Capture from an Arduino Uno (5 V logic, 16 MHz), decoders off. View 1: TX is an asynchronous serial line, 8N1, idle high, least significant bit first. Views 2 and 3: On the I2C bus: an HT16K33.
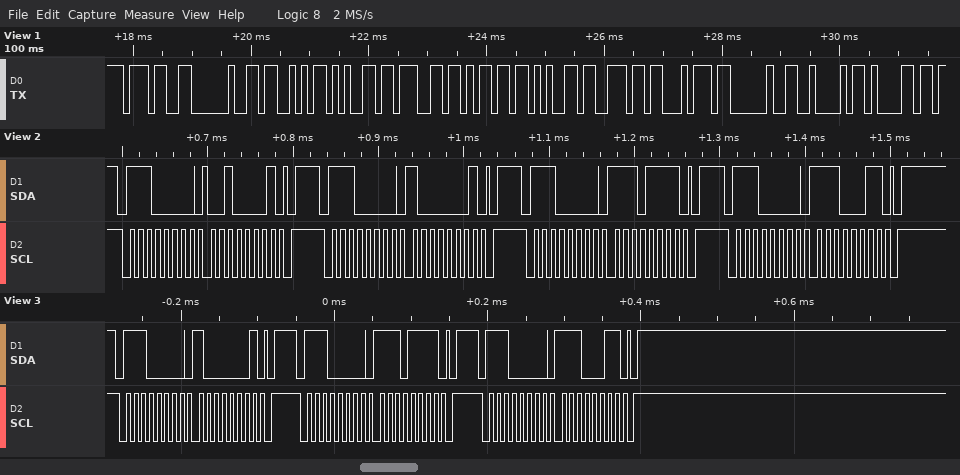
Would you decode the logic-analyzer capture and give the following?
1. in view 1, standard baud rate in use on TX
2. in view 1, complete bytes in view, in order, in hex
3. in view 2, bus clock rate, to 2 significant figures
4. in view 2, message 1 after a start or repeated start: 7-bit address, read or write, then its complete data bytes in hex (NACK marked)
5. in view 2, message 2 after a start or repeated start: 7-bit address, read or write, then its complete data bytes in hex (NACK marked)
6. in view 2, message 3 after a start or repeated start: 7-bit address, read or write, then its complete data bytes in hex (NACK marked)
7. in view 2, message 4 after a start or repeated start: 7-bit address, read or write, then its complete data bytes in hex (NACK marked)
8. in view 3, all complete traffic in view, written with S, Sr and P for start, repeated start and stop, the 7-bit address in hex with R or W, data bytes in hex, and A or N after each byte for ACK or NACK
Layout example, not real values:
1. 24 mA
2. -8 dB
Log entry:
1. 9600 baud
2. 37 20 53 65 67 6D 65 6E 74 20 42 61
3. 100 kHz
4. 0x70 write: 21
5. 0x70 write: 81
6. 0x70 write: EF
7. 0x70 write: E3
8. S 70W A 81 A P S 70W A EF A P S 70W A E3 A P
